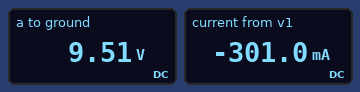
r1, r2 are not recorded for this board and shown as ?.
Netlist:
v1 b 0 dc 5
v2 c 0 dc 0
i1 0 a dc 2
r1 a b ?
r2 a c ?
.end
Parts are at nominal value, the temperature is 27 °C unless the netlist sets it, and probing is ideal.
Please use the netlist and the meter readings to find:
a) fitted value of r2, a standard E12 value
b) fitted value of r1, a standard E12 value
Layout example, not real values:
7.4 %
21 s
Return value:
5.6 Ω
15 Ω
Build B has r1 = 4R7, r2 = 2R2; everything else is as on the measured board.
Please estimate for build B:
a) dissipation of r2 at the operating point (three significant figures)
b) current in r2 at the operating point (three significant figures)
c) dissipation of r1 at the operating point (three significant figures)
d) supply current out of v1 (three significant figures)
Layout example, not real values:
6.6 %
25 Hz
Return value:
9.58 W
2.09 A
35.5 mW
87.0 mA
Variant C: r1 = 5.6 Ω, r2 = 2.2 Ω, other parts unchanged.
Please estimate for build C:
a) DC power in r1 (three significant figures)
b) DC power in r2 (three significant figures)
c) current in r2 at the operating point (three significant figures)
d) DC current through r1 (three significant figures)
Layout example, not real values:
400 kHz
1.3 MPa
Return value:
33.1 mW
9.49 W
2.08 A
76.9 mA
